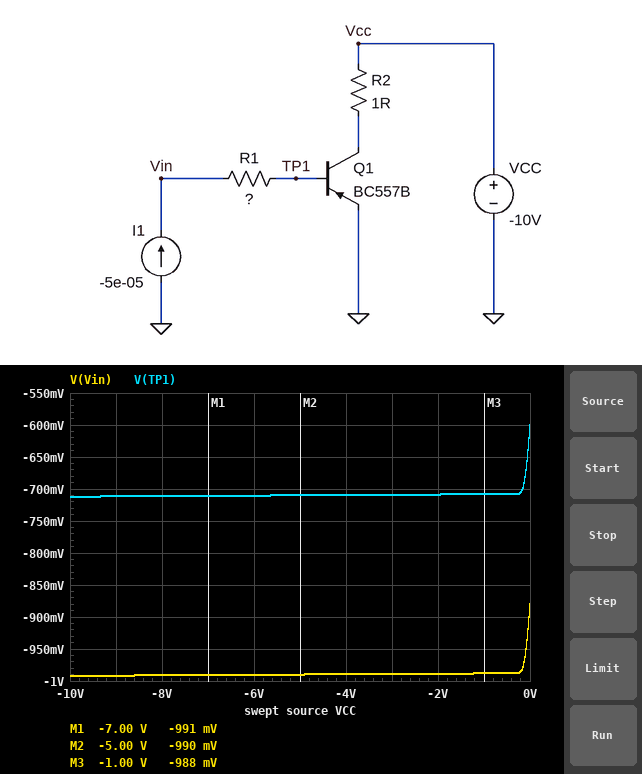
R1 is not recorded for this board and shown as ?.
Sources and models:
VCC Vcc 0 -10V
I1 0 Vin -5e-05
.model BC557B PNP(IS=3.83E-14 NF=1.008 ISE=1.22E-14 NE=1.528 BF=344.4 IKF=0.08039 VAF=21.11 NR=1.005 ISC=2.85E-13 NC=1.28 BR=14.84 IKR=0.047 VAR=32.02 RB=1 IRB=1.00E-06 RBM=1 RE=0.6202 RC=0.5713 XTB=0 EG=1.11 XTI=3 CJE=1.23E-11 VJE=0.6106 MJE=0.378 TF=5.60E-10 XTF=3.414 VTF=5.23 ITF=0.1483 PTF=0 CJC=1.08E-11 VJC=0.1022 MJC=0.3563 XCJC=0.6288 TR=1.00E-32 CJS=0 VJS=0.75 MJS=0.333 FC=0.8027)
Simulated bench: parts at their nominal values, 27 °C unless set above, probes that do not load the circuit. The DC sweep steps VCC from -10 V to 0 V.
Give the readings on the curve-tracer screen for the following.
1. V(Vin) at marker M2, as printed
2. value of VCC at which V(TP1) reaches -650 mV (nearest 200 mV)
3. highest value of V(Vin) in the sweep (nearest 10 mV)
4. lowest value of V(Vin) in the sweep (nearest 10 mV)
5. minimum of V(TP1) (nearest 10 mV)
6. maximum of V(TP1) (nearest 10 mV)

-990 mV
0 V
-880 mV
-990 mV
-710 mV
-600 mV
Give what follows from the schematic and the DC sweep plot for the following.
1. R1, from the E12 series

5.6 kΩ
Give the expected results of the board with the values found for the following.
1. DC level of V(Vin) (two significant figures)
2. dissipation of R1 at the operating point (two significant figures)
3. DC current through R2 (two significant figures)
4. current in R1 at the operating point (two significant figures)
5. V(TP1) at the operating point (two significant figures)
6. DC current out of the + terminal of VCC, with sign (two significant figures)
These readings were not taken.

-990 mV
14 µW
20 mA
50 µA
-710 mV
-20 mA
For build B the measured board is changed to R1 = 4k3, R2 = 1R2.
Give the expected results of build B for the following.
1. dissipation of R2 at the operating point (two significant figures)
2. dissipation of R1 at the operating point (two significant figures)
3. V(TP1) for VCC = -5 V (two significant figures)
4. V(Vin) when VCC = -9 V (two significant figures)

500 µW
11 µW
-710 mV
-930 mV
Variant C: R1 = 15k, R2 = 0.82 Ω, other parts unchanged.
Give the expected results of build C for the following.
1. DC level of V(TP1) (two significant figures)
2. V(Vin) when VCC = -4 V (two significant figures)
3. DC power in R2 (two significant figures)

-710 mV
-1.5 V
340 µW
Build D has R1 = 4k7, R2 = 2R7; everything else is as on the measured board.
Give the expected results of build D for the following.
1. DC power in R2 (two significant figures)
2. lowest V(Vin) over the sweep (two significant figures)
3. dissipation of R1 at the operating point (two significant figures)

1.1 mW
-950 mV
12 µW
